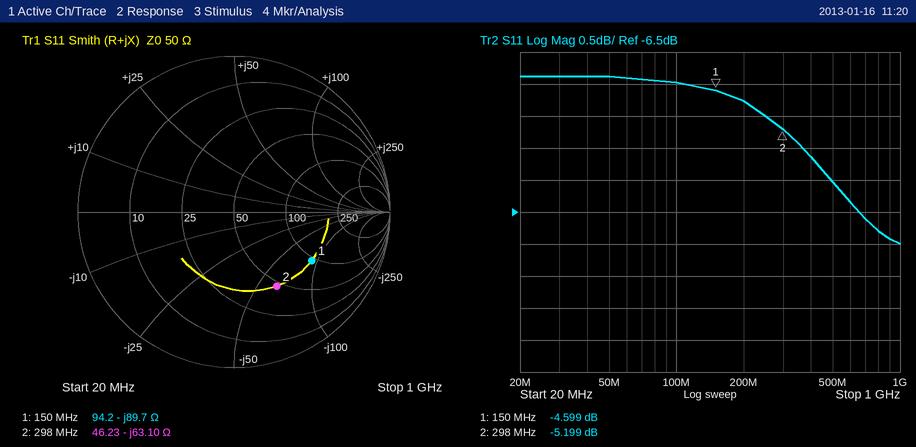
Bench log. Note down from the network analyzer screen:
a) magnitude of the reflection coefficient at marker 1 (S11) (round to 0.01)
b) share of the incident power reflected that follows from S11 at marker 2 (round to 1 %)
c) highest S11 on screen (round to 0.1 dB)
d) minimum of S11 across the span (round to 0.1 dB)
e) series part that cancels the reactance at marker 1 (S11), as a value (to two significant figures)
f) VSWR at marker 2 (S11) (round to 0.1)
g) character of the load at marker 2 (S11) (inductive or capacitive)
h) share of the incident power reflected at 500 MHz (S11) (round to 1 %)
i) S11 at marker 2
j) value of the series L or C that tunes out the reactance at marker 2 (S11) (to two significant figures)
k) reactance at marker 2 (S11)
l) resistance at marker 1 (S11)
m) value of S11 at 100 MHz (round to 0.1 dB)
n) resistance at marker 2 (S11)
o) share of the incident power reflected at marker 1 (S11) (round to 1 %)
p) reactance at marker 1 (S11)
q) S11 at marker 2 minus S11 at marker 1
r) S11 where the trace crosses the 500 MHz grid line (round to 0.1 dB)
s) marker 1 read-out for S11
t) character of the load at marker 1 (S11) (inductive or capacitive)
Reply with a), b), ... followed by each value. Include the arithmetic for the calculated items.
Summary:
a) 0.59
b) 10^(-5.199/10) ≈ 30 %
c) -4.4 dB
d) -7.0 dB
e) L = 89.7 Ω/(2π × 150 MHz) ≈ 95 nH
f) 3.4
g) capacitive
h) 10^(-6/10) ≈ 25 %
i) -5.199 dB
j) L = 63.1 Ω/(2π × 298 MHz) ≈ 34 nH
k) -63.10 Ω
l) 94.2 Ω
m) -4.5 dB
n) 46.23 Ω
o) 10^(-4.599/10) ≈ 35 %
p) -89.7 Ω
q) -5.199 − (-4.599) = -0.600 dB
r) -6.0 dB
s) -4.599 dB
t) capacitive
